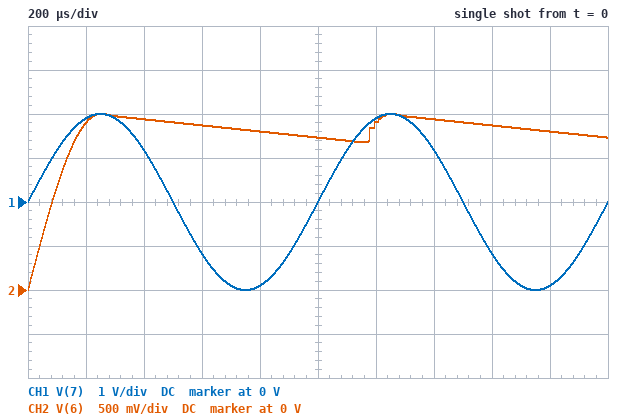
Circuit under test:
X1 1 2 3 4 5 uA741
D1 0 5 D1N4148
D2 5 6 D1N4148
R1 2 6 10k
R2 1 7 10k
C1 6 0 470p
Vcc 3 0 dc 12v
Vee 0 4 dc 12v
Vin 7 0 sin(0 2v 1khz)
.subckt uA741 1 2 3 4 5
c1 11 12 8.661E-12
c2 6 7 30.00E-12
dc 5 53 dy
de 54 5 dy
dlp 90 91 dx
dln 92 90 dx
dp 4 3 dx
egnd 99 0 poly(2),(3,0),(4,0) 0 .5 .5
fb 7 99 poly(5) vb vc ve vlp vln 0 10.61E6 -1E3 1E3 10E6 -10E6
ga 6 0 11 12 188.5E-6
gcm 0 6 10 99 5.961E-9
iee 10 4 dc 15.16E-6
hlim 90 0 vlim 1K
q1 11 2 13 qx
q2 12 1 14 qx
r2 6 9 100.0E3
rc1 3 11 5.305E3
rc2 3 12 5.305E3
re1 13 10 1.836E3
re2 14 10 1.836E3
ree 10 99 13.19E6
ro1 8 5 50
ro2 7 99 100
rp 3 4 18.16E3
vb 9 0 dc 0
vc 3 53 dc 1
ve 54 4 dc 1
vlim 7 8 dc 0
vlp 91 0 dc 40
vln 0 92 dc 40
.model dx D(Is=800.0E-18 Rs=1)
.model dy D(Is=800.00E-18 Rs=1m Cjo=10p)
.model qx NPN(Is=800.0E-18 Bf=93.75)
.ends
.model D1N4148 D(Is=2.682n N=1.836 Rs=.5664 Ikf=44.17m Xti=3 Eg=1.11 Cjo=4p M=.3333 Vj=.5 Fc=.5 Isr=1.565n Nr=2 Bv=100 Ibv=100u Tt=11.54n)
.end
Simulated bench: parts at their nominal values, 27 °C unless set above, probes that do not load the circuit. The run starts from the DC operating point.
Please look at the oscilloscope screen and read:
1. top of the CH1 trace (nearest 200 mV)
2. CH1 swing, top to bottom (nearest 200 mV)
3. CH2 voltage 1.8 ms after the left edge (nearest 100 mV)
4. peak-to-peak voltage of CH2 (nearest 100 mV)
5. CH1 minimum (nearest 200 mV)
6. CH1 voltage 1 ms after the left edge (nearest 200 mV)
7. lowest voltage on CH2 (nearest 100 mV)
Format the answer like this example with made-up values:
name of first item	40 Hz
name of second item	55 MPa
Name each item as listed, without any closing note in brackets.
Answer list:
top of the CH1 trace	2.0 V
CH1 swing, top to bottom	4.0 V
CH2 voltage 1.8 ms after the left edge	1.8 V
peak-to-peak voltage of CH2	2.0 V
CH1 minimum	-2.0 V
CH1 voltage 1 ms after the left edge	0 V
lowest voltage on CH2	0 V
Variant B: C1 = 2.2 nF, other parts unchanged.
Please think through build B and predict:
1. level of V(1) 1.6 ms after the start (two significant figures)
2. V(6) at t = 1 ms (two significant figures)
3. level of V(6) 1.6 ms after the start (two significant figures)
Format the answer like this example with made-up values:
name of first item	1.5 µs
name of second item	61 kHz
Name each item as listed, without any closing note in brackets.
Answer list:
level of V(1) 1.6 ms after the start	-1.2 V
V(6) at t = 1 ms	1.9 V
level of V(6) 1.6 ms after the start	2.0 V
